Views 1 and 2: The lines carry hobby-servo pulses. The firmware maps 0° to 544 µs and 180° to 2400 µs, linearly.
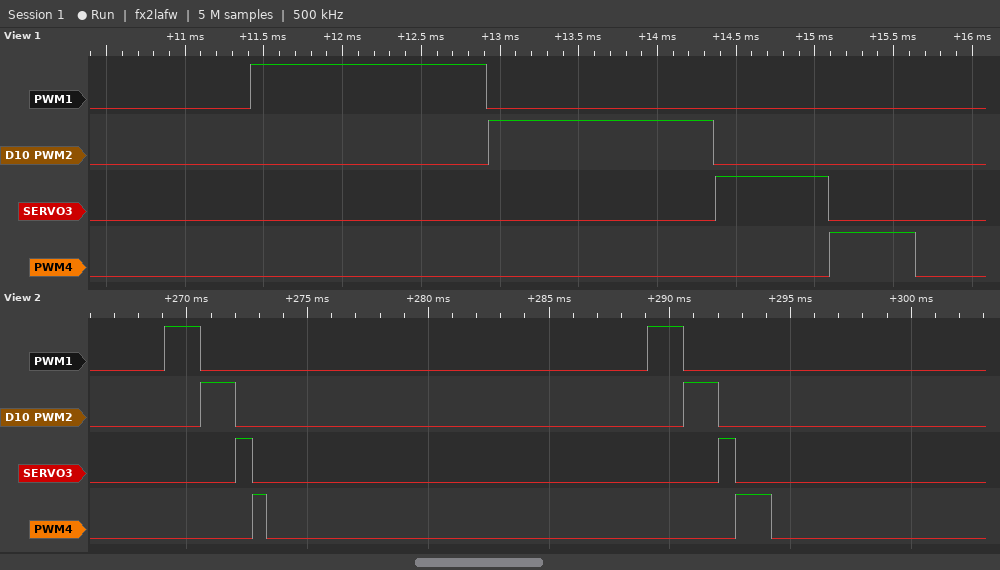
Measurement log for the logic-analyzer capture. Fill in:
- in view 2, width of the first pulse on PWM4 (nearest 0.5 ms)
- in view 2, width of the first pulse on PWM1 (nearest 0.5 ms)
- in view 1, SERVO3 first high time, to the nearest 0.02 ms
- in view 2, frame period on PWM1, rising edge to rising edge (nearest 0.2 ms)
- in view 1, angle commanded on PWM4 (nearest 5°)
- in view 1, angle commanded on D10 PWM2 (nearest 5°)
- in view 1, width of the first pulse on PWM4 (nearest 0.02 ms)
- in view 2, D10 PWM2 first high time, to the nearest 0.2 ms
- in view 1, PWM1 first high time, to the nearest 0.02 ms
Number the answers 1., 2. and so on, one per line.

1. 0.5 ms
2. 1.5 ms
3. 0.72 ms
4. 20.0 ms
5. 0°
6. 85°
7. 0.54 ms
8. 1.4 ms
9. 1.50 ms
